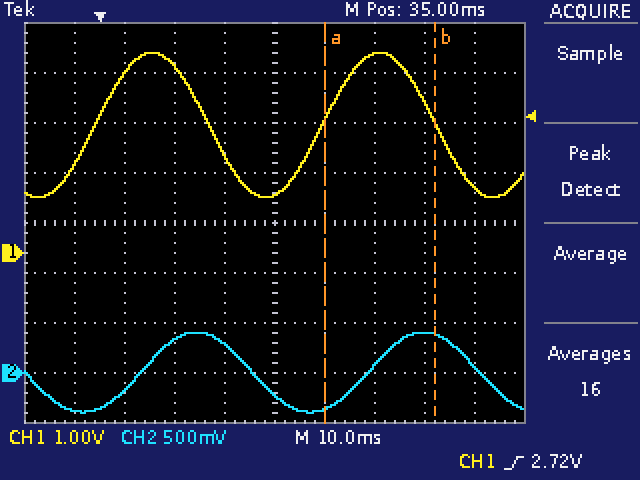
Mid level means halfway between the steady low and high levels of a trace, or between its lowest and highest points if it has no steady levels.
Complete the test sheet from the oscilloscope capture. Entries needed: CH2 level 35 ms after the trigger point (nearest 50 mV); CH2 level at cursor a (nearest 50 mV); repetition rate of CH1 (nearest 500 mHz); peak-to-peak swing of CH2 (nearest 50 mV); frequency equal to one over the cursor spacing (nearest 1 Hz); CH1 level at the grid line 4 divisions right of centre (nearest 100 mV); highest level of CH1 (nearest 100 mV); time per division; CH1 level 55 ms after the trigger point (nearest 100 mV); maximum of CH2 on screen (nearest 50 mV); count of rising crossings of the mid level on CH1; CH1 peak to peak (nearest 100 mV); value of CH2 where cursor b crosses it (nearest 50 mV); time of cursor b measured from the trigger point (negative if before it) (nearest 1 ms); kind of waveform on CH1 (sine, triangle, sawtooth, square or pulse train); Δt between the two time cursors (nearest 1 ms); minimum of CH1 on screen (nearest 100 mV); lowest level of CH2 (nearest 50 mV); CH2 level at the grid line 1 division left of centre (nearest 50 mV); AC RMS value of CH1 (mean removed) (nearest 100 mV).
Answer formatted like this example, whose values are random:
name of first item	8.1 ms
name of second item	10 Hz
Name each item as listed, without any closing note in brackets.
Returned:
CH2 level 35 ms after the trigger point	-200 mV
CH2 level at cursor a	-350 mV
repetition rate of CH1	22.0 Hz
peak-to-peak swing of CH2	800 mV
frequency equal to one over the cursor spacing	45 Hz
CH1 level at the grid line 4 divisions right of centre	1.3 V
highest level of CH1	4.0 V
time per division	10 ms
CH1 level 55 ms after the trigger point	4.0 V
maximum of CH2 on screen	400 mV
count of rising crossings of the mid level on CH1	2
CH1 peak to peak	2.9 V
value of CH2 where cursor b crosses it	400 mV
time of cursor b measured from the trigger point (negative if before it)	+67 ms
kind of waveform on CH1	sine
Δt between the two time cursors	22 ms
minimum of CH1 on screen	1.1 V
lowest level of CH2	-400 mV
CH2 level at the grid line 1 division left of centre	300 mV
AC RMS value of CH1 (mean removed)	1.0 V
